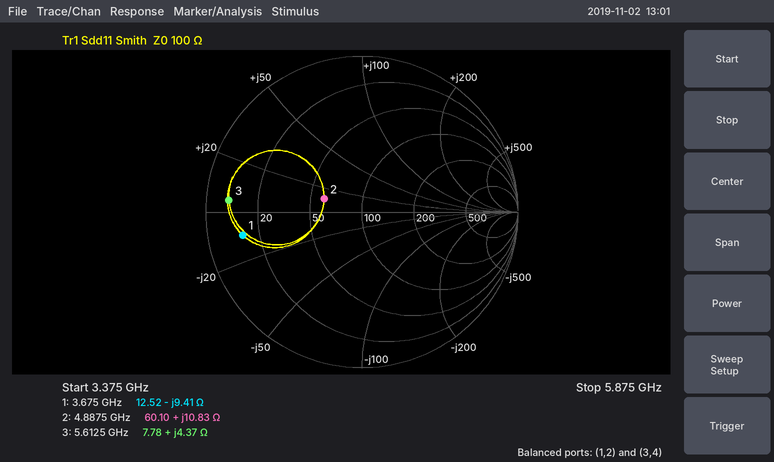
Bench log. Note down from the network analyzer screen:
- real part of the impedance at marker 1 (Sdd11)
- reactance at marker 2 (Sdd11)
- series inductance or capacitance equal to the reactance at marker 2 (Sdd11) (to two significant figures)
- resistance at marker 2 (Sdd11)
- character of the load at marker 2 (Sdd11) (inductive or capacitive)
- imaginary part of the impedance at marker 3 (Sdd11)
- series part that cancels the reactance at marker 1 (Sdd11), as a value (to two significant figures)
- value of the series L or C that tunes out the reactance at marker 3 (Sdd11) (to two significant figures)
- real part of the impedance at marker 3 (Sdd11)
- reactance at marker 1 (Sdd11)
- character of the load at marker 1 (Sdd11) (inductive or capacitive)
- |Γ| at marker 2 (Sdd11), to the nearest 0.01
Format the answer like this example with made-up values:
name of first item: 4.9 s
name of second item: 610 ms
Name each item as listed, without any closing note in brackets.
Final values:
real part of the impedance at marker 1: 12.52 Ω
reactance at marker 2: +10.83 Ω
series inductance or capacitance equal to the reactance at marker 2 (Sdd11): 350 pH
resistance at marker 2: 60.10 Ω
character of the load at marker 2 (Sdd11): inductive
imaginary part of the impedance at marker 3: +4.37 Ω
series part that cancels the reactance at marker 1 (Sdd11), as a value: 410 pH
value of the series L or C that tunes out the reactance at marker 3 (Sdd11): 6.5 pF
real part of the impedance at marker 3: 7.78 Ω
reactance at marker 1: -9.41 Ω
character of the load at marker 1 (Sdd11): capacitive
|Γ| at marker 2 (Sdd11), to the nearest 0.01: 0.26
